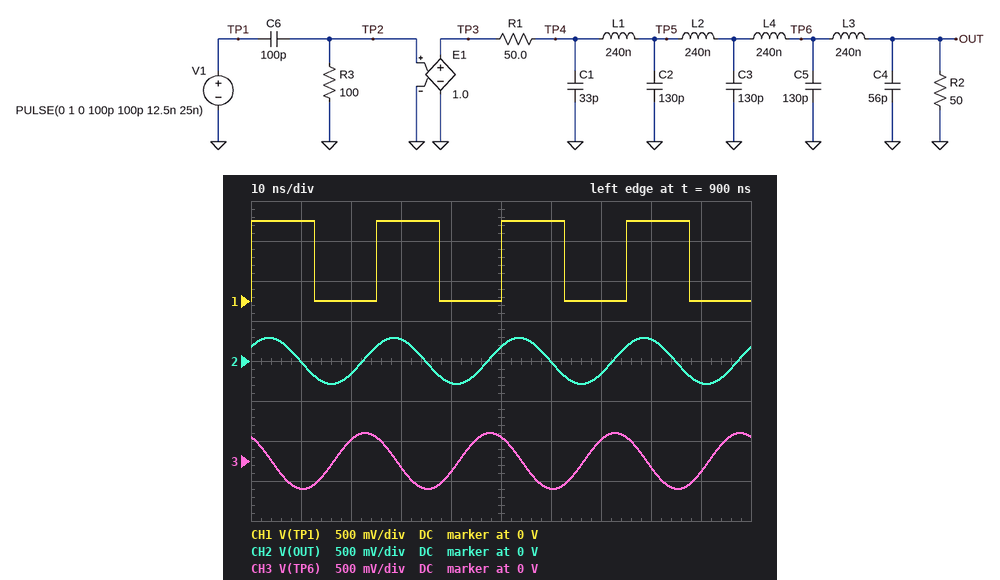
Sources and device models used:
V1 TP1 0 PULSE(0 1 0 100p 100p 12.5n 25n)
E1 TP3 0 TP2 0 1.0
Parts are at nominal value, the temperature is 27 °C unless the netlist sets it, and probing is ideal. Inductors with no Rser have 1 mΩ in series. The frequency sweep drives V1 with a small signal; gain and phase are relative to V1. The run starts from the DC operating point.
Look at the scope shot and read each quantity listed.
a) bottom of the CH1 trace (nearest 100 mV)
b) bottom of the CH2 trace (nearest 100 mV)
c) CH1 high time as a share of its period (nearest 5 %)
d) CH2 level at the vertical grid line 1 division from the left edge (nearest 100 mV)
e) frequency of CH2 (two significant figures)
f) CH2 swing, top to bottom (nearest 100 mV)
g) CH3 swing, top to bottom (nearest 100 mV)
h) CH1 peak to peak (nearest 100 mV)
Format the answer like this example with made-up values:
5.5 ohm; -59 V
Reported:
0 V; -300 mV; 50 %; 0 V; 40 MHz; 600 mV; 700 mV; 1.0 V
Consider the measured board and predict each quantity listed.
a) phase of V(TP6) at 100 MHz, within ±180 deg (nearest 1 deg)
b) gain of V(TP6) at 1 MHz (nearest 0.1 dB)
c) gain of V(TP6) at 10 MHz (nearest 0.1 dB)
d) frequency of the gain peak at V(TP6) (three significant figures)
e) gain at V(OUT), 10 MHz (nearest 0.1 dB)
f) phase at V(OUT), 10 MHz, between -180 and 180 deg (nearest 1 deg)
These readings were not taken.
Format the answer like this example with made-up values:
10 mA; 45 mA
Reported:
156 deg; -30.1 dB; -11.6 dB; 52.0 MHz; -11.6 dB; -20 deg
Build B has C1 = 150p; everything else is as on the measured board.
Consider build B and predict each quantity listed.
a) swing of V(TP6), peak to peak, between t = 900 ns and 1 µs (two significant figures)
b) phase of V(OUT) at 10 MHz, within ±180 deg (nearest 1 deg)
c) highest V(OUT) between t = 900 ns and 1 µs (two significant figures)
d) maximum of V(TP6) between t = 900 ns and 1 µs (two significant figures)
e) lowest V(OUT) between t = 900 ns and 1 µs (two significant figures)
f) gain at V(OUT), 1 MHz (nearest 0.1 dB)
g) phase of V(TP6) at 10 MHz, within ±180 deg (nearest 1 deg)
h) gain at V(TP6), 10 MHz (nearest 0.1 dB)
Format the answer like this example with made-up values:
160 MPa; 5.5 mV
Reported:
650 mV; -29 deg; 270 mV; 320 mV; -270 mV; -30.1 dB; -11 deg; -11.7 dB
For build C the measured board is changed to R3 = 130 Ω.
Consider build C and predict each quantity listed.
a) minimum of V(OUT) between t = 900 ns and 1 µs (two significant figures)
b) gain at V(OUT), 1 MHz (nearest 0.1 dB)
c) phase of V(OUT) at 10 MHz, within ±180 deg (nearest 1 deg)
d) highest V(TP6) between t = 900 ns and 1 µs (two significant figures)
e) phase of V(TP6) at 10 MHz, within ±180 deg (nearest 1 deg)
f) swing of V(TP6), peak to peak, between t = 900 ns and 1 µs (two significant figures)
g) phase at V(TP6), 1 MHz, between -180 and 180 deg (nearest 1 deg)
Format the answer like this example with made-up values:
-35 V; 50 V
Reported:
-300 mV; -27.8 dB; -27 deg; 360 mV; -9 deg; 720 mV; 79 deg
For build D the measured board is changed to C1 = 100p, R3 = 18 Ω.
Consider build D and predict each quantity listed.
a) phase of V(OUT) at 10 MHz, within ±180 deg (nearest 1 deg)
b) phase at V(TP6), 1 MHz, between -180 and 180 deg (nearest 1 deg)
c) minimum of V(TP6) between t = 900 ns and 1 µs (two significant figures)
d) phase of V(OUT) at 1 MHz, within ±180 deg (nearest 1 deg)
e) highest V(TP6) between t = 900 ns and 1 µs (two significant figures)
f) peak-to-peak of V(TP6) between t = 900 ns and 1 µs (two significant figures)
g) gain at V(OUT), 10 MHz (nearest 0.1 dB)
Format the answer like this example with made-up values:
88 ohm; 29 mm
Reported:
1 deg; 83 deg; -160 mV; 81 deg; 160 mV; 310 mV; -25.1 dB
